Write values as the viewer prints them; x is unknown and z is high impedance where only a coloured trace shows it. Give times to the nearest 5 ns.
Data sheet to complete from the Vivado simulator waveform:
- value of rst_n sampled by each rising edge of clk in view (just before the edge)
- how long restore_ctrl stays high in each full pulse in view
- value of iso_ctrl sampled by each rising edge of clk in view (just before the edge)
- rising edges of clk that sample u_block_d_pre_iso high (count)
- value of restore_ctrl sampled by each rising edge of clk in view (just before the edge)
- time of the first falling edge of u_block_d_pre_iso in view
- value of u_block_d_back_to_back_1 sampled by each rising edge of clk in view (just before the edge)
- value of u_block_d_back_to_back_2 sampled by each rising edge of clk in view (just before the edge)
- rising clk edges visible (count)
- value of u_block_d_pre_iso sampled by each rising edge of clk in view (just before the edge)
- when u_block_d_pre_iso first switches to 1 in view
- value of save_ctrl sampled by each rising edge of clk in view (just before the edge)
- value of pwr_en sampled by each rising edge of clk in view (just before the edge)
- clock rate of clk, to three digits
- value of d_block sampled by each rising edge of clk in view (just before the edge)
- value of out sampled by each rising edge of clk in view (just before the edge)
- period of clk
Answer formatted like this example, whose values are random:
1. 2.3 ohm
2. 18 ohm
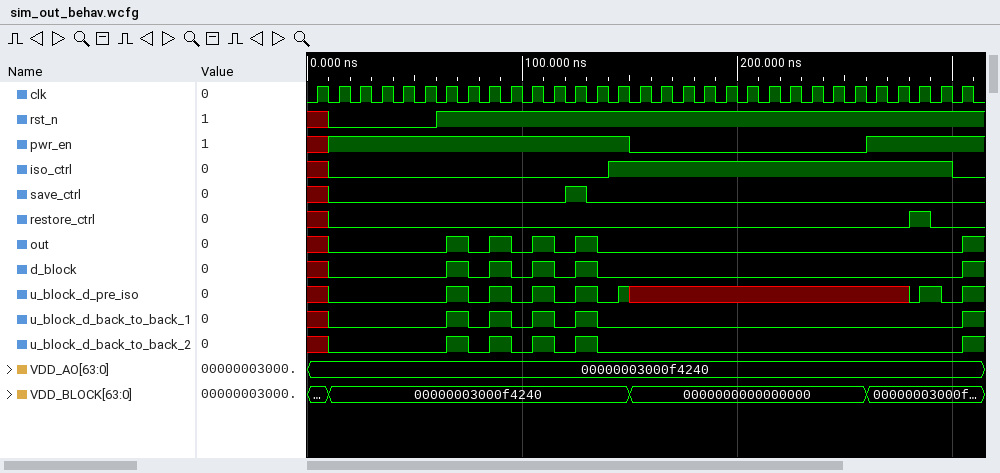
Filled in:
1. x 0 0 0 0 0 1 1 1 1 1 1 1 1 1 1 1 1 1 1 1 1 1 1 1 1 1 1 1 1 1
2. 10 ns
3. x 0 0 0 0 0 0 0 0 0 0 0 0 0 1 1 1 1 1 1 1 1 1 1 1 1 1 1 1 1 0
4. 5
5. x 0 0 0 0 0 0 0 0 0 0 0 0 0 0 0 0 0 0 0 0 0 0 0 0 0 0 0 1 0 0
6. 75 ns
7. x 0 0 0 0 0 0 1 0 1 0 1 0 1 0 0 0 0 0 0 0 0 0 0 0 0 0 0 0 0 0
8. x 0 0 0 0 0 0 1 0 1 0 1 0 1 0 0 0 0 0 0 0 0 0 0 0 0 0 0 0 0 0
9. 31
10. x 0 0 0 0 0 0 1 0 1 0 1 0 1 0 x x x x x x x x x x x x x 0 1 0
11. 65 ns
12. x 0 0 0 0 0 0 0 0 0 0 0 1 0 0 0 0 0 0 0 0 0 0 0 0 0 0 0 0 0 0
13. x 1 1 1 1 1 1 1 1 1 1 1 1 1 1 0 0 0 0 0 0 0 0 0 0 0 1 1 1 1 1
14. 100 MHz
15. x 0 0 0 0 0 0 1 0 1 0 1 0 1 0 0 0 0 0 0 0 0 0 0 0 0 0 0 0 0 0
16. x 0 0 0 0 0 0 1 0 1 0 1 0 1 0 0 0 0 0 0 0 0 0 0 0 0 0 0 0 0 0
17. 10 ns
